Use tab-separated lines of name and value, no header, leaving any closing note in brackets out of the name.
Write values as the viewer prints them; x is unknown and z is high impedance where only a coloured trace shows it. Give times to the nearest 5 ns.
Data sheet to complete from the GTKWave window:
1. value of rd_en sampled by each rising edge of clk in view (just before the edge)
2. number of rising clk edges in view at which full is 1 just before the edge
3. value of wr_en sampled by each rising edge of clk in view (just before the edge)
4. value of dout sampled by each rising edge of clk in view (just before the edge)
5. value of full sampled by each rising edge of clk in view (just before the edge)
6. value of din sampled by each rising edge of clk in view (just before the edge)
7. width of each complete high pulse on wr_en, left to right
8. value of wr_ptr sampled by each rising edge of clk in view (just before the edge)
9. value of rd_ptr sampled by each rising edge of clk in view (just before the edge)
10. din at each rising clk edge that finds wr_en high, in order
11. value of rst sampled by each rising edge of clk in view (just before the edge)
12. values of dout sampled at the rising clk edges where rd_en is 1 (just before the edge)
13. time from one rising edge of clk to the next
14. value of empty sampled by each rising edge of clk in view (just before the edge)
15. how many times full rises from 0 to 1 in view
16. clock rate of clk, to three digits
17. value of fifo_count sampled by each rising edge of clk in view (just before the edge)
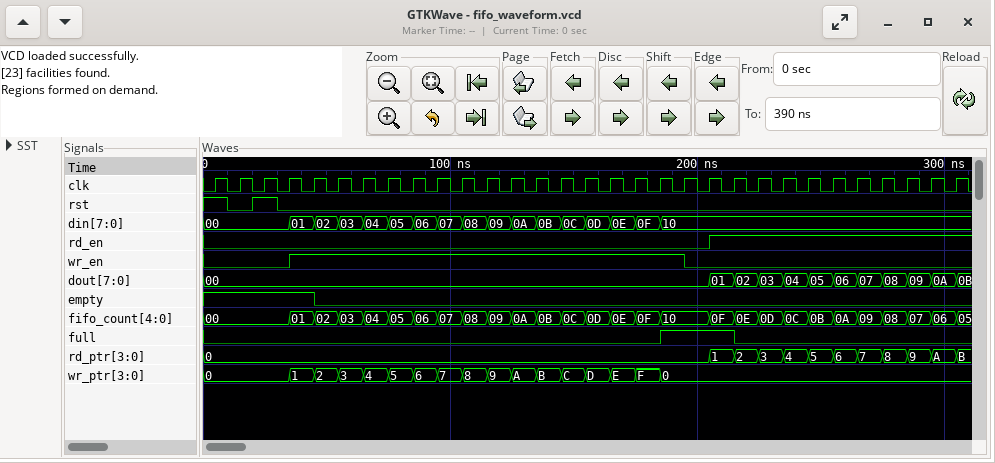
value of rd_en sampled by each rising edge of clk in view	0 0 0 0 0 0 0 0 0 0 0 0 0 0 0 0 0 0 0 0 0 1 1 1 1 1 1 1 1 1 1
number of rising clk edges in view at which full is 1 just before the edge	3
value of wr_en sampled by each rising edge of clk in view	0 0 0 0 1 1 1 1 1 1 1 1 1 1 1 1 1 1 1 1 0 0 0 0 0 0 0 0 0 0 0
value of dout sampled by each rising edge of clk in view	00, 00, 00, 00, 00, 00, 00, 00, 00, 00, 00, 00, 00, 00, 00, 00, 00, 00, 00, 00, 00, 01, 02, 03, 04, 05, 06, 07, 08, 09, 0A
value of full sampled by each rising edge of clk in view	0 0 0 0 0 0 0 0 0 0 0 0 0 0 0 0 0 0 0 1 1 1 0 0 0 0 0 0 0 0 0
value of din sampled by each rising edge of clk in view	00, 00, 00, 00, 01, 02, 03, 04, 05, 06, 07, 08, 09, 0A, 0B, 0C, 0D, 0E, 0F, 10, 10, 10, 10, 10, 10, 10, 10, 10, 10, 10, 10
width of each complete high pulse on wr_en, left to right	160 ns
value of wr_ptr sampled by each rising edge of clk in view	0, 0, 0, 0, 1, 2, 3, 4, 5, 6, 7, 8, 9, A, B, C, D, E, F, 0, 0, 0, 0, 0, 0, 0, 0, 0, 0, 0, 0
value of rd_ptr sampled by each rising edge of clk in view	0, 0, 0, 0, 0, 0, 0, 0, 0, 0, 0, 0, 0, 0, 0, 0, 0, 0, 0, 0, 0, 1, 2, 3, 4, 5, 6, 7, 8, 9, A
din at each rising clk edge that finds wr_en high, in order	01, 02, 03, 04, 05, 06, 07, 08, 09, 0A, 0B, 0C, 0D, 0E, 0F, 10
value of rst sampled by each rising edge of clk in view	1 0 1 0 0 0 0 0 0 0 0 0 0 0 0 0 0 0 0 0 0 0 0 0 0 0 0 0 0 0 0
values of dout sampled at the rising clk edges where rd_en is 1	01, 02, 03, 04, 05, 06, 07, 08, 09, 0A
time from one rising edge of clk to the next	10 ns
value of empty sampled by each rising edge of clk in view	1 1 1 1 1 0 0 0 0 0 0 0 0 0 0 0 0 0 0 0 0 0 0 0 0 0 0 0 0 0 0
how many times full rises from 0 to 1 in view	1
clock rate of clk, to three digits	100 MHz
value of fifo_count sampled by each rising edge of clk in view	00, 00, 00, 00, 01, 02, 03, 04, 05, 06, 07, 08, 09, 0A, 0B, 0C, 0D, 0E, 0F, 10, 10, 0F, 0E, 0D, 0C, 0B, 0A, 09, 08, 07, 06
